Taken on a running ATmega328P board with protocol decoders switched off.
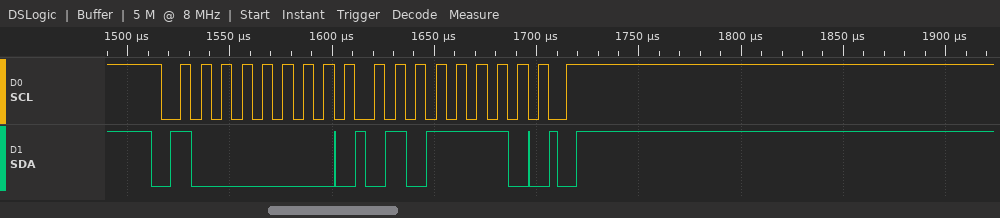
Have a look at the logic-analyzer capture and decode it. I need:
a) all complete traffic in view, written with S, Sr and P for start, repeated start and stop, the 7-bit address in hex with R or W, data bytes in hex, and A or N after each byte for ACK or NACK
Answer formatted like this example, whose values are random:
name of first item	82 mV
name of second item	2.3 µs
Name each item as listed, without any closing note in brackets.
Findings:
all complete traffic in view, written with S, Sr and P for start, repeated start and stop, the 7-bit address in hex with R or W, data bytes in hex, and A or N after each byte for ACK or NACK	S 40W A 5E A P
